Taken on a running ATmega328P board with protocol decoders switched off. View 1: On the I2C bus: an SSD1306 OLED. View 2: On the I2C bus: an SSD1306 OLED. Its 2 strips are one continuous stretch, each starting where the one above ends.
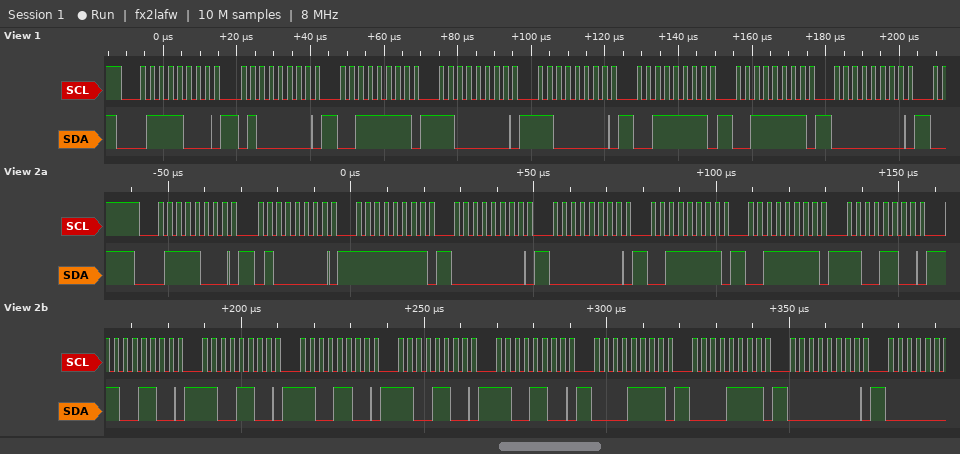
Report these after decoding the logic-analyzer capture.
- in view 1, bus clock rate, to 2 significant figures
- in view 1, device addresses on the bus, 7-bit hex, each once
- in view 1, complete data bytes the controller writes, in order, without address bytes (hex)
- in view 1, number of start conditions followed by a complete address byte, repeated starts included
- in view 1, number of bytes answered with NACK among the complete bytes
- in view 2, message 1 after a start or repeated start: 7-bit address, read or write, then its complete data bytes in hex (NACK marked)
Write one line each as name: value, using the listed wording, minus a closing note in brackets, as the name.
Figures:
in view 1, bus clock rate, to 2 significant figures: 400 kHz
in view 1, device addresses on the bus, 7-bit hex, each once: 0x3C
in view 1, complete data bytes the controller writes, in order, without address bytes: 40 3F C0 C0 3F 3F 00
in view 1, number of start conditions followed by a complete address byte, repeated starts included: 1
in view 1, number of bytes answered with NACK among the complete bytes: 0
in view 2, message 1 after a start or repeated start: 7-bit address, read or write, then its complete data bytes in hex: 0x3C write: 40 FF 00 00 3F 3F CC CC CC CC CC CC 0F 0F 00
